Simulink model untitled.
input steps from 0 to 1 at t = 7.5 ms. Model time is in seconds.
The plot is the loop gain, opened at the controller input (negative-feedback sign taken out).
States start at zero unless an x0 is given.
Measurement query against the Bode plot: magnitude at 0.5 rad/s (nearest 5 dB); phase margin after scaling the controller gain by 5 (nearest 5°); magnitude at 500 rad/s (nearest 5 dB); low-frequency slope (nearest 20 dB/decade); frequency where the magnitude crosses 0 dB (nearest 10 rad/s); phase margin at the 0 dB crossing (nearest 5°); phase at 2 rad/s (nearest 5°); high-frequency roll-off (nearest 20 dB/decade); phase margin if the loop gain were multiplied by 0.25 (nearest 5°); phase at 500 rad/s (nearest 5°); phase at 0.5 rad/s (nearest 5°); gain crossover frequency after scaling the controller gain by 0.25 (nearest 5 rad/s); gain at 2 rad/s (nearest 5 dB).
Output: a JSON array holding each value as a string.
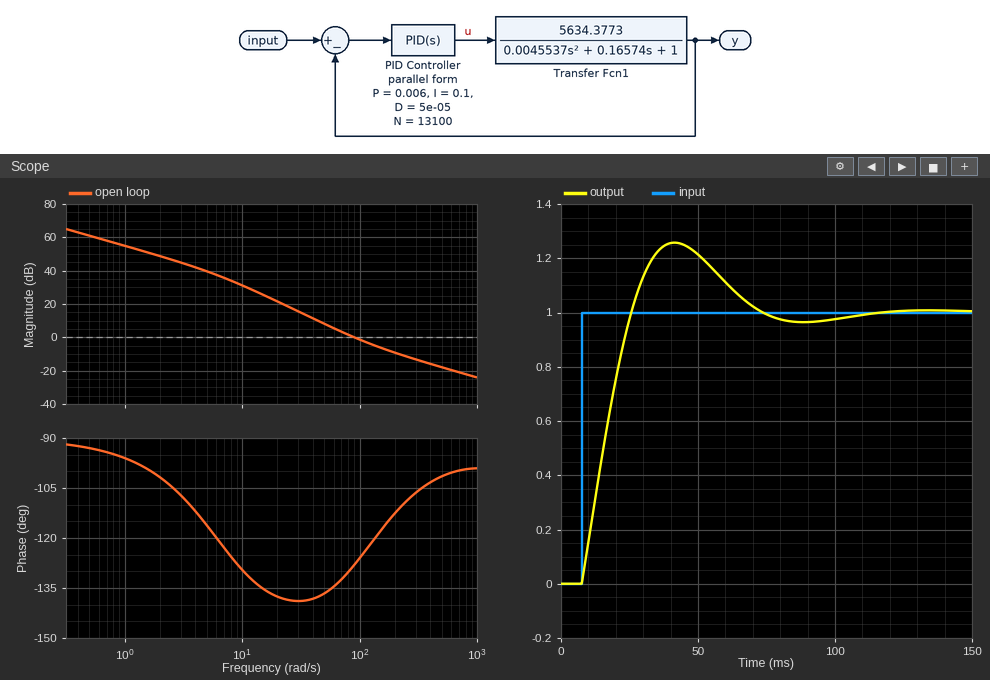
["60 dB", "75°", "-20 dB", "-20 dB/decade", "90 rad/s", "50°", "-100°", "-20 dB/decade", "40°", "-100°", "-95°", "40 rad/s", "50 dB"]
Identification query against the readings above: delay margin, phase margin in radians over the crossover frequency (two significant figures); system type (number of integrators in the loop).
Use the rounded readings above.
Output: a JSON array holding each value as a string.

["0.0097 s", "1"]
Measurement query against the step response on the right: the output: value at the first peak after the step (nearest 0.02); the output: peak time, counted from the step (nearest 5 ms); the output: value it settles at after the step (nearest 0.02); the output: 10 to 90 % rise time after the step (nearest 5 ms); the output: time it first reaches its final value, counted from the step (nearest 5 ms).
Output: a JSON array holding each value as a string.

["1.26", "35 ms", "1.00", "15 ms", "20 ms"]
